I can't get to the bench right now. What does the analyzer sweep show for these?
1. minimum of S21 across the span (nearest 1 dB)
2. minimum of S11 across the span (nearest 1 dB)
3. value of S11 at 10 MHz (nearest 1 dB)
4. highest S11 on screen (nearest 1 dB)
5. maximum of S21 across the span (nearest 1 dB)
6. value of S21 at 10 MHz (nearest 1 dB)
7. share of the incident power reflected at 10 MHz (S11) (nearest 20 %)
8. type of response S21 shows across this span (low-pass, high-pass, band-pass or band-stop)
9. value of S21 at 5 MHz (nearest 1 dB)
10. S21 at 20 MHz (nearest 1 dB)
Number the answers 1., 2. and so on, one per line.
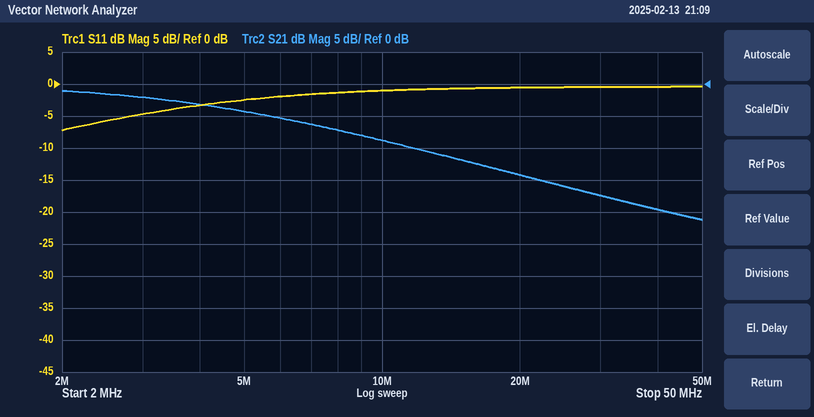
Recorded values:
1. -21 dB
2. -7 dB
3. -1 dB
4. 0 dB
5. -1 dB
6. -9 dB
7. 80 %
8. low-pass
9. -4 dB
10. -14 dB
